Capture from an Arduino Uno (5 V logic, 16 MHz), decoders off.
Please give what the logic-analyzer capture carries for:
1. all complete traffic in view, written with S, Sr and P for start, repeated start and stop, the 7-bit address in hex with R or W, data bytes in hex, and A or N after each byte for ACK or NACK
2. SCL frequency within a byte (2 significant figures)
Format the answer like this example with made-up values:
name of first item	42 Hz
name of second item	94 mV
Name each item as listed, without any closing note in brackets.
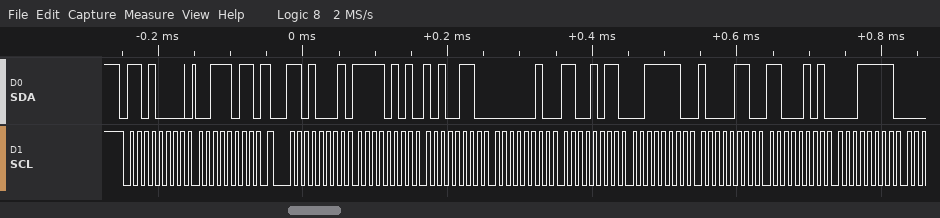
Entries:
all complete traffic in view, written with S, Sr and P for start, repeated start and stop, the 7-bit address in hex with R or W, data bytes in hex, and A or N after each byte for ACK or NACK	S 68W A 3B A Sr 68R A F5 A A6 A 02 A CB A 3E A 86 A C5 A 1F A
SCL frequency within a byte	100 kHz
